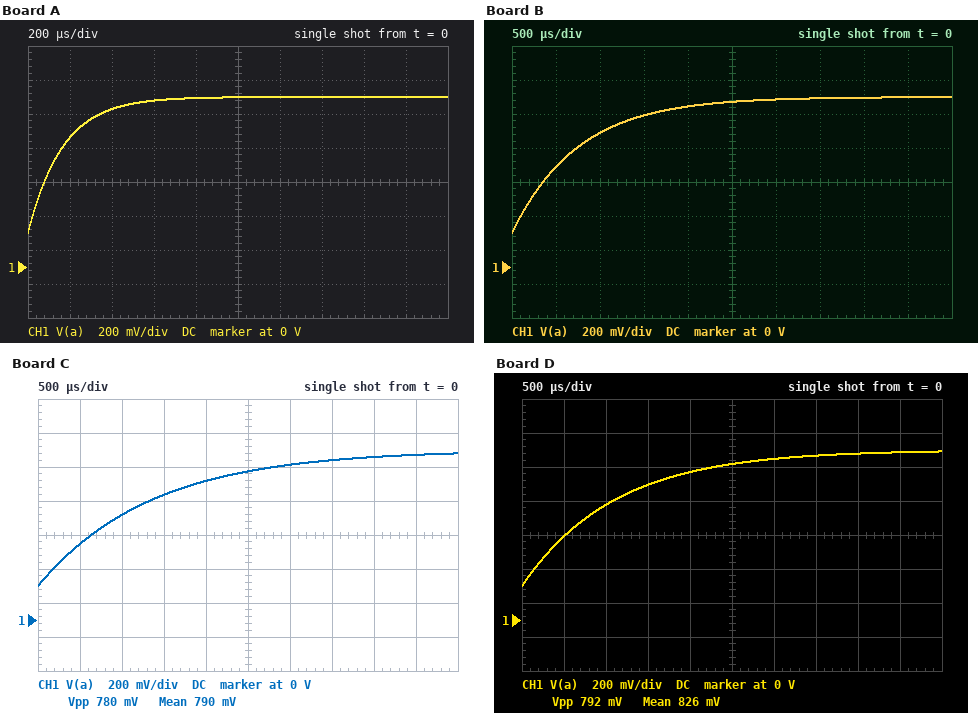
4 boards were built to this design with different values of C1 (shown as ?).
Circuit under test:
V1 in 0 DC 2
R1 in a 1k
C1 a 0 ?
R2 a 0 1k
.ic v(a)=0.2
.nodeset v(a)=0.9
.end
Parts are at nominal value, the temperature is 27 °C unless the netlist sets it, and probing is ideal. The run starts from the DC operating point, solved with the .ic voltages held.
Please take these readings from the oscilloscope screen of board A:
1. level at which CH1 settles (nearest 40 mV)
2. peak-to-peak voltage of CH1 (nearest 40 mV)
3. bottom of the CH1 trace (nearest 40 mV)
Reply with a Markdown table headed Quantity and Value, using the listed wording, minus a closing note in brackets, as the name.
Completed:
| Quantity | Value |
|---|---|
| level at which CH1 settles | 1.00 V |
| peak-to-peak voltage of CH1 | 800 mV |
| bottom of the CH1 trace | 200 mV |
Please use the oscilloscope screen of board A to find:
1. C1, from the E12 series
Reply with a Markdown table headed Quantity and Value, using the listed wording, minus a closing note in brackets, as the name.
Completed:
| Quantity | Value |
|---|---|
| C1, from the E12 series | 330 nF |
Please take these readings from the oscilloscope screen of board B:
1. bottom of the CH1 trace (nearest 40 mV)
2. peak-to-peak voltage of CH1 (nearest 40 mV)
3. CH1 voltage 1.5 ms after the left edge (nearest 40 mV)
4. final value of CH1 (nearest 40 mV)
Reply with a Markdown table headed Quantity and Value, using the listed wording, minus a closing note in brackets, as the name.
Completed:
| Quantity | Value |
|---|---|
| bottom of the CH1 trace | 200 mV |
| peak-to-peak voltage of CH1 | 800 mV |
| CH1 voltage 1.5 ms after the left edge | 880 mV |
| final value of CH1 | 1.00 V |
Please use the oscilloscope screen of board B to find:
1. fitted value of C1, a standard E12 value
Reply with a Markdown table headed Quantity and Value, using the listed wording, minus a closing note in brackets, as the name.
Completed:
| Quantity | Value |
|---|---|
| fitted value of C1, a standard E12 value | 1.5 µF |
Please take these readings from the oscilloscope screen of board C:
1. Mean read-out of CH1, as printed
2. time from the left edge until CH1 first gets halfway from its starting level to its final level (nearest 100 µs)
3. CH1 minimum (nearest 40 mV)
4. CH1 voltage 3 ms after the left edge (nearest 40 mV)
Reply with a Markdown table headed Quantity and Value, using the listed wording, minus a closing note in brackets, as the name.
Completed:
| Quantity | Value |
|---|---|
| Mean read-out of CH1, as printed | 790 mV |
| time from the left edge until CH1 first gets halfway from its starting level to its final level | 900 µs |
| CH1 minimum | 200 mV |
| CH1 voltage 3 ms after the left edge | 920 mV |
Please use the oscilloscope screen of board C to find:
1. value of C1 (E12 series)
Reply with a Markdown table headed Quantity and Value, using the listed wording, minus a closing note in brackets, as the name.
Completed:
| Quantity | Value |
|---|---|
| value of C1 | 2.7 µF |
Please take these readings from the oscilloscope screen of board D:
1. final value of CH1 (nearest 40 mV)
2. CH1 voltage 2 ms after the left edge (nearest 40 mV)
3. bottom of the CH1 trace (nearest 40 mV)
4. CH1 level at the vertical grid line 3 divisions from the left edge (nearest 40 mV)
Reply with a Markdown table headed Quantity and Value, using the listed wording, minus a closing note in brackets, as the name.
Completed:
| Quantity | Value |
|---|---|
| final value of CH1 | 1.00 V |
| CH1 voltage 2 ms after the left edge | 880 mV |
| bottom of the CH1 trace | 200 mV |
| CH1 level at the vertical grid line 3 divisions from the left edge | 800 mV |
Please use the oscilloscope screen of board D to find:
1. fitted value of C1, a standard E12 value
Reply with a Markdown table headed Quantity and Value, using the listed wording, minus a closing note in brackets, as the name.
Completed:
| Quantity | Value |
|---|---|
| fitted value of C1, a standard E12 value | 2.2 µF |
